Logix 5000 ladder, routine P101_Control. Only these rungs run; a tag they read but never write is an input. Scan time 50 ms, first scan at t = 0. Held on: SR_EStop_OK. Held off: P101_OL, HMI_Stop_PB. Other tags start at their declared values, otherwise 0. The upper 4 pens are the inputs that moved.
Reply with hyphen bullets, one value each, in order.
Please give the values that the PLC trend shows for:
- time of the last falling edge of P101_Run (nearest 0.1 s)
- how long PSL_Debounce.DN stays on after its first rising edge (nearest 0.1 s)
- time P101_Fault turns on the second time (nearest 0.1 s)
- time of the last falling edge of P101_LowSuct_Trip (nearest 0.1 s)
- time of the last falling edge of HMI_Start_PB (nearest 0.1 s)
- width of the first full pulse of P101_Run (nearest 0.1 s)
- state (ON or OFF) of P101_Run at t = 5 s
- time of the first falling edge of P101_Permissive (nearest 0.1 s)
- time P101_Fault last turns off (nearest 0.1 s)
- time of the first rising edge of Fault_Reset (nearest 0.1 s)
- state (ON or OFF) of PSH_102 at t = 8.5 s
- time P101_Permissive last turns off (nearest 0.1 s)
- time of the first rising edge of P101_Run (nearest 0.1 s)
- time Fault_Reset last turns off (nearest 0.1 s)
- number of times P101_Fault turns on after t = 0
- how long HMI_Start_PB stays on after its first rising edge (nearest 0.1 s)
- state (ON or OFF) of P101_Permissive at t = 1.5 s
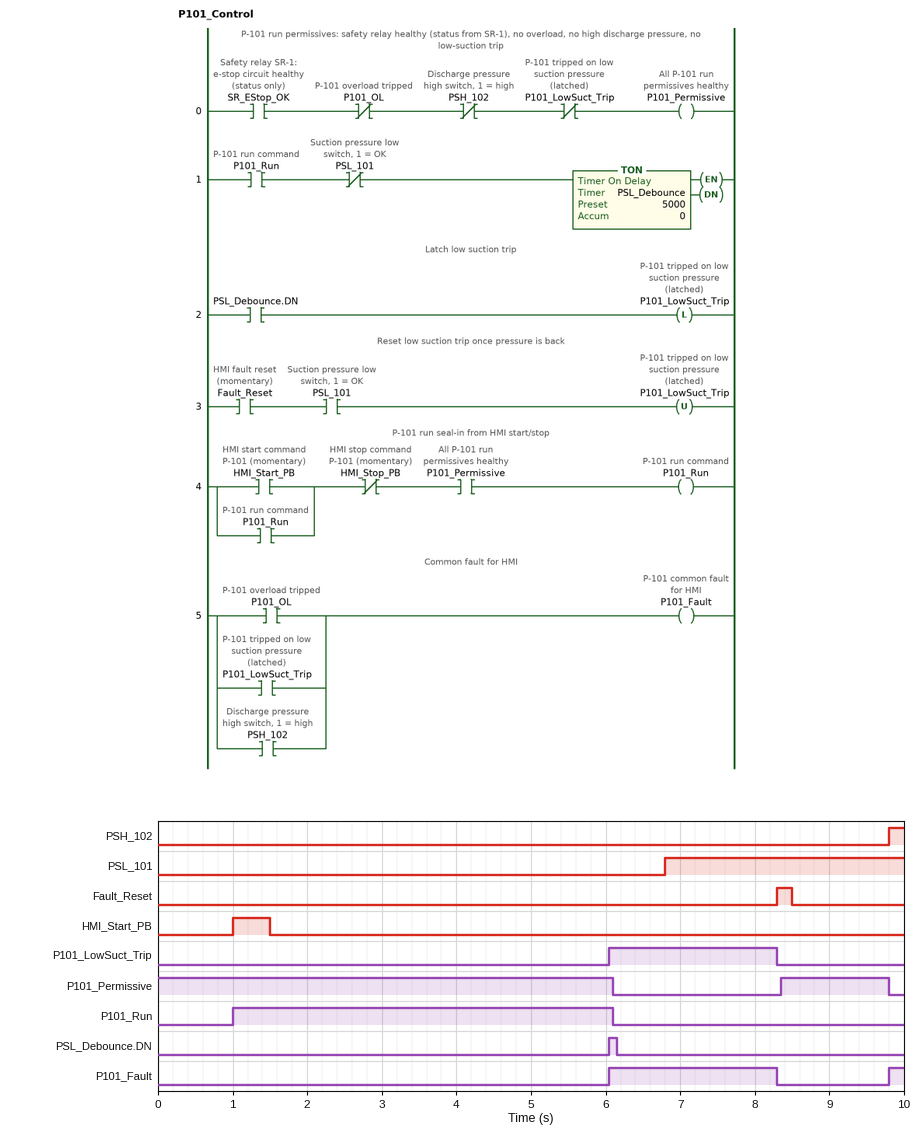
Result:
- 6.1 s
- 0.1 s
- 9.8 s
- 8.3 s
- 1.5 s
- 5.1 s
- ON
- 6.1 s
- 8.3 s
- 8.3 s
- OFF
- 9.8 s
- 1.0 s
- 8.5 s
- 2
- 0.5 s
- ON
